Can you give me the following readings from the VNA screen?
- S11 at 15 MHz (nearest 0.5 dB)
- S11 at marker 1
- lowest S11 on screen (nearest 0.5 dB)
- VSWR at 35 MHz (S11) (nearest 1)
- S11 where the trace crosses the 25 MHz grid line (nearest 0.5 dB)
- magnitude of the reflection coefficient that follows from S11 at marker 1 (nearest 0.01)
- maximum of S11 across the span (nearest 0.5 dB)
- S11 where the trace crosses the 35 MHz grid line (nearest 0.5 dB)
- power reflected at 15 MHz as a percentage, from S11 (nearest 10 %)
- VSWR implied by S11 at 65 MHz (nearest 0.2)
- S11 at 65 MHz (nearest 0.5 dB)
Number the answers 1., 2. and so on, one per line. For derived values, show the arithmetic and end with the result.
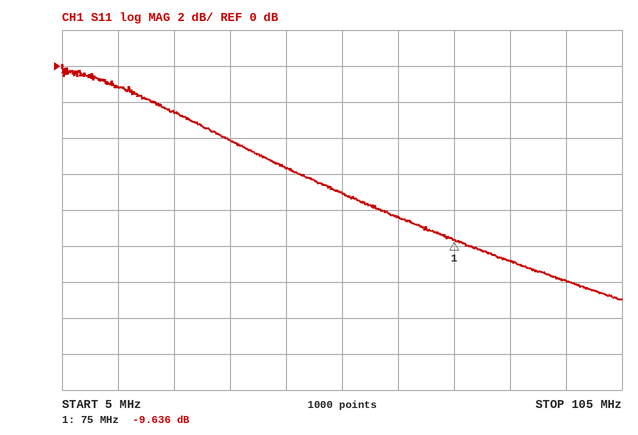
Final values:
1. -1.0 dB
2. -9.636 dB
3. -13.0 dB
4. |Γ| = 10^(-4/20) = 0.6310; VSWR = (1 + 0.6310)/(1 − 0.6310) ≈ 4
5. -2.5 dB
6. 10^(-9.636/20) ≈ 0.33
7. 0.0 dB
8. -4.0 dB
9. 10^(-1/10) ≈ 79.4 %, so 80 % to the nearest 10 %
10. |Γ| = 10^(-8.5/20) = 0.3758; VSWR = (1 + 0.3758)/(1 − 0.3758) ≈ 2.2
11. -8.5 dB
